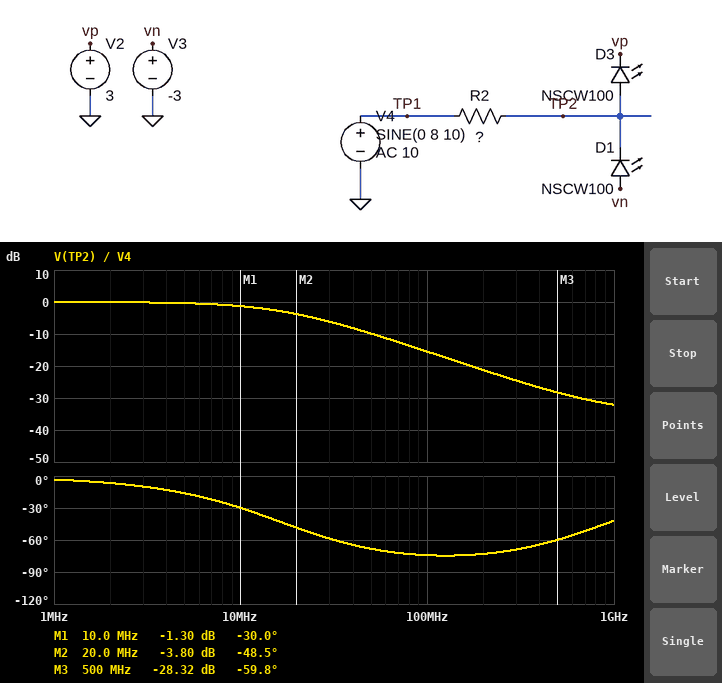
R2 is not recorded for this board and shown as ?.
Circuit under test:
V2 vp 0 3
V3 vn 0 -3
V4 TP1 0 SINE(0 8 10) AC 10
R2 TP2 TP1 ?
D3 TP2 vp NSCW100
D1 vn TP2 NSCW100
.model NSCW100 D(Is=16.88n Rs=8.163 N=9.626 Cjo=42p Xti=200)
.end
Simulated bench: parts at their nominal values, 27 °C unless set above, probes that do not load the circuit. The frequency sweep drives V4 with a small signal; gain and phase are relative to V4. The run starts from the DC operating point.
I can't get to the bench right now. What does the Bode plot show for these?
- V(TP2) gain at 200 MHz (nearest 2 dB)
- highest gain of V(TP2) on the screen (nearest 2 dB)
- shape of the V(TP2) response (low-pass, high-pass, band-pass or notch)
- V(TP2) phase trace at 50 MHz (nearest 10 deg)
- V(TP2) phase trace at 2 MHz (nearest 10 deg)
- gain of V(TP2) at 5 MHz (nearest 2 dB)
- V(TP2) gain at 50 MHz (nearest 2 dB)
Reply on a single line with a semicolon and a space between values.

-22 dB; 0 dB; low-pass; -70 deg; -10 deg; 0 dB; -10 dB
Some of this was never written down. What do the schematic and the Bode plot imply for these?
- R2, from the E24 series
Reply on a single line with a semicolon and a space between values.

220 Ω
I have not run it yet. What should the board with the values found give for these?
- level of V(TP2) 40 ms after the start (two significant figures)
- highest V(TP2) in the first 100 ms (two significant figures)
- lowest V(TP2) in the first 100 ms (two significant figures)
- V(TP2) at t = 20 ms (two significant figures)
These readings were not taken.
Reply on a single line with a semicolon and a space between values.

4.7 V; 6.3 V; -6.3 V; 6.2 V
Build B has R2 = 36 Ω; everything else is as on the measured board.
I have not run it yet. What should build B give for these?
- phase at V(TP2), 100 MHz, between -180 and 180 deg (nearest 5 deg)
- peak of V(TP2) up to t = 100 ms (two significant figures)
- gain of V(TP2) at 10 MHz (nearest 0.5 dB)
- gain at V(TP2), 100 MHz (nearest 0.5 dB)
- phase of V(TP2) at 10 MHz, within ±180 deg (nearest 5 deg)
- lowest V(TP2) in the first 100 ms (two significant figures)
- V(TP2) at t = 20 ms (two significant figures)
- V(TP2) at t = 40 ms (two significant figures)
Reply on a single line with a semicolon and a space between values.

-40 deg; 6.9 V; 0 dB; -3.0 dB; -5 deg; -6.9 V; 6.7 V; 4.7 V
